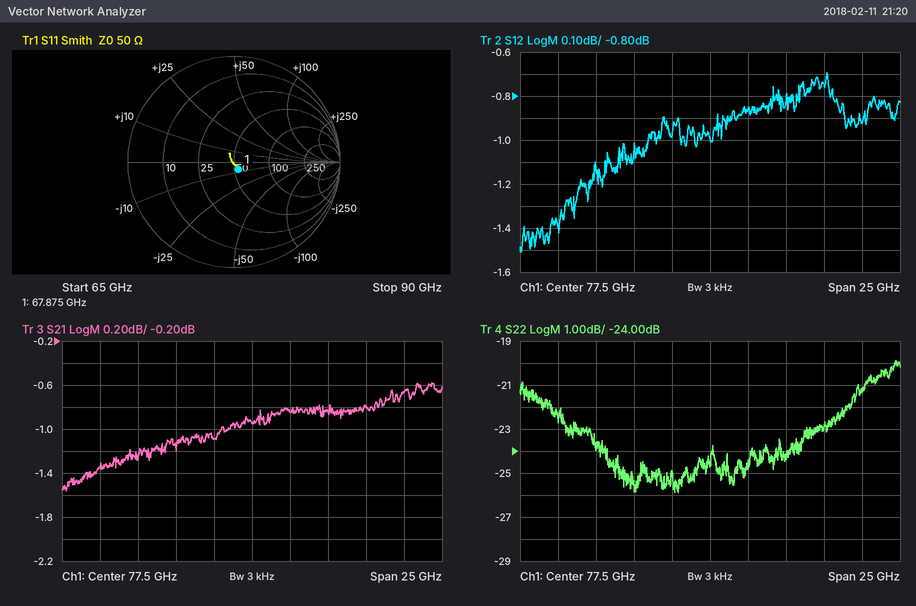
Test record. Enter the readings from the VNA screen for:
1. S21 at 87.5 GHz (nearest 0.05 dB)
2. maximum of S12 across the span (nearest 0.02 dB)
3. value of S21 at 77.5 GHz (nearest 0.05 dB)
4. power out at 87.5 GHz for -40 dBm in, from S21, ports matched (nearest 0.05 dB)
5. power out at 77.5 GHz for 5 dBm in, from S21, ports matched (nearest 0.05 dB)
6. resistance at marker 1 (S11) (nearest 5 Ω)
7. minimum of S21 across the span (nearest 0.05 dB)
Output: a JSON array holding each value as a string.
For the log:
["-0.65 dB", "-0.70 dB", "-0.95 dB", "-40.65 dBm", "4.05 dBm", "55 Ω", "-1.55 dB"]
